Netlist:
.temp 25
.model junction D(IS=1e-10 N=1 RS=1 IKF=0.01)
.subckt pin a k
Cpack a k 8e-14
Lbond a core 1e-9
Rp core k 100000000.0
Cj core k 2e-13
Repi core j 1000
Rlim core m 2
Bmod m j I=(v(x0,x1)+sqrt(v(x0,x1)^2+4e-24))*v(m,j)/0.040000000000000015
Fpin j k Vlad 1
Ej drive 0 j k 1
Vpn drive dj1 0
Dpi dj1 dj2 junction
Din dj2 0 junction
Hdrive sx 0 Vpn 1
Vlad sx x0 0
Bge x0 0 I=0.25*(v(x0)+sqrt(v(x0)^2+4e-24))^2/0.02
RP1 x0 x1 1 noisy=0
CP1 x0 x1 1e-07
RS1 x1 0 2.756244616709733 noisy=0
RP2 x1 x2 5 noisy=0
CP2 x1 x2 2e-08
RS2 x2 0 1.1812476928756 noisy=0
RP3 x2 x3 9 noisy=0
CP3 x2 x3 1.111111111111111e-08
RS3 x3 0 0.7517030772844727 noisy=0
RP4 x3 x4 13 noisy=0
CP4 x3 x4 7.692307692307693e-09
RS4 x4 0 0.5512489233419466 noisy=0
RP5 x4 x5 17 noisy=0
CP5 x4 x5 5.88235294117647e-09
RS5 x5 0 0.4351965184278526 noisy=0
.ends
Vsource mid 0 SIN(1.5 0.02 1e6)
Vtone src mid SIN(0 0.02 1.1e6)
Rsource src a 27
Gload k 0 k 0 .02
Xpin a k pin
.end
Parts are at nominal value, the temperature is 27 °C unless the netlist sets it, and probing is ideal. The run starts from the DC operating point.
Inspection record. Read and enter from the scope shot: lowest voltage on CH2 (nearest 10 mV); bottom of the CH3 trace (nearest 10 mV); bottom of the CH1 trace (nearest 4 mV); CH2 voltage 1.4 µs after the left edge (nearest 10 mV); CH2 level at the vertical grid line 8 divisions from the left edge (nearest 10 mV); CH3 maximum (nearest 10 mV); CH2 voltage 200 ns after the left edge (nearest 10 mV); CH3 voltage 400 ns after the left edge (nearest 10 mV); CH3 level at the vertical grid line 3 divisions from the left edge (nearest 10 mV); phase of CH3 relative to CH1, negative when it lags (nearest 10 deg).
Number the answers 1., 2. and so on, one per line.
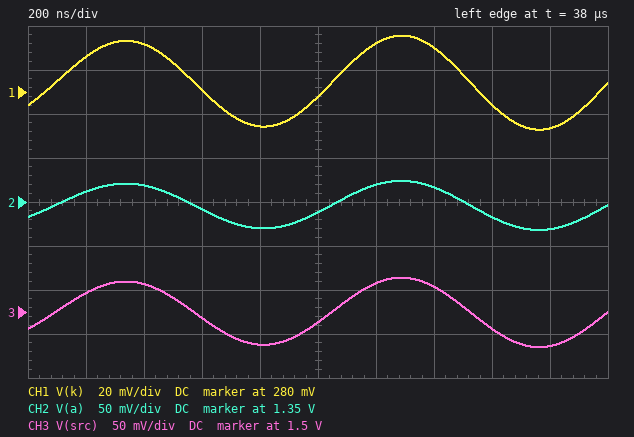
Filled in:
1. 1.32 V
2. 1.46 V
3. 264 mV
4. 1.37 V
5. 1.33 V
6. 1.54 V
7. 1.36 V
8. 1.53 V
9. 1.49 V
10. 0 deg
